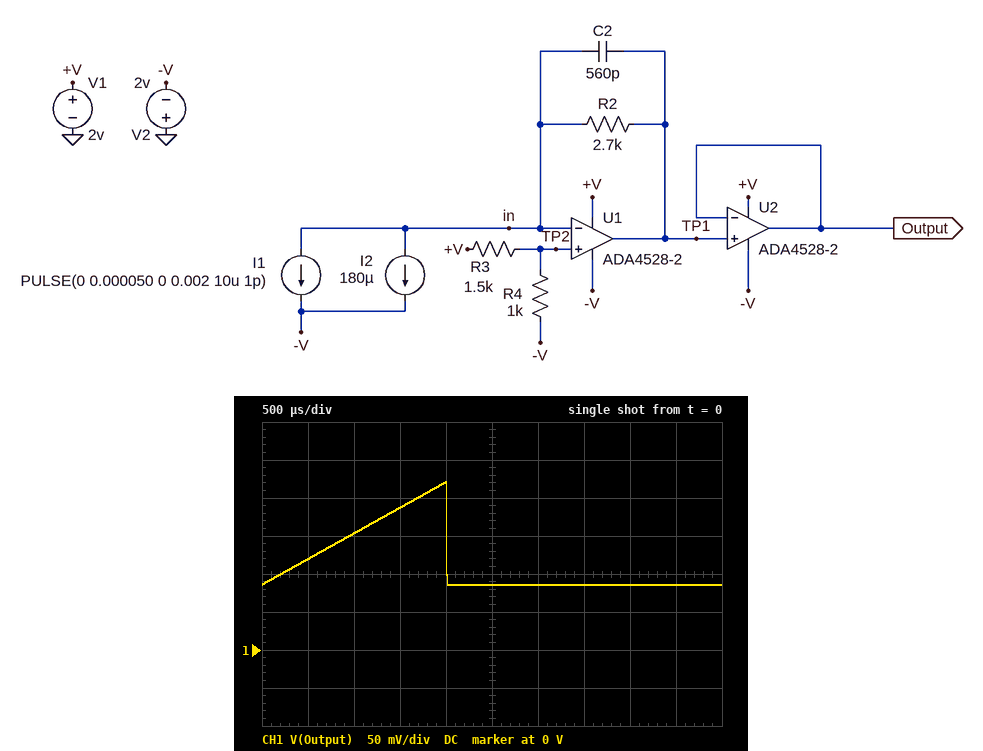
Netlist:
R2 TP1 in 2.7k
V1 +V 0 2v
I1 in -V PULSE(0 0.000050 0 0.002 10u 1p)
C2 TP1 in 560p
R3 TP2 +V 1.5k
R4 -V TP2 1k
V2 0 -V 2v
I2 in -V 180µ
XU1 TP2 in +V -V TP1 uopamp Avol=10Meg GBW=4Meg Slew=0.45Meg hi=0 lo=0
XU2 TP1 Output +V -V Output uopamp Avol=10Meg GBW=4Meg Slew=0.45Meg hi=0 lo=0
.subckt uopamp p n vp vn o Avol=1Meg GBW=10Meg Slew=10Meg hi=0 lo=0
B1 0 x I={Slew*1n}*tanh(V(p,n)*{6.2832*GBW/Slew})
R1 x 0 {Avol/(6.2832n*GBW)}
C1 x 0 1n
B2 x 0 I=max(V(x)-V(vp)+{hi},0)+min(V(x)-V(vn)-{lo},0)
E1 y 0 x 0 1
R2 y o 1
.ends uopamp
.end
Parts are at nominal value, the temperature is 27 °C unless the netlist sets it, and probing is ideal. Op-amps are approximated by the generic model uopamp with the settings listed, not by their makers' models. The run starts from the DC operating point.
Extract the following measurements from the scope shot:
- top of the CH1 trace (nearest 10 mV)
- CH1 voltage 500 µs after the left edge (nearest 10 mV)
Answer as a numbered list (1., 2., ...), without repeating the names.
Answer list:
1. 220 mV
2. 120 mV
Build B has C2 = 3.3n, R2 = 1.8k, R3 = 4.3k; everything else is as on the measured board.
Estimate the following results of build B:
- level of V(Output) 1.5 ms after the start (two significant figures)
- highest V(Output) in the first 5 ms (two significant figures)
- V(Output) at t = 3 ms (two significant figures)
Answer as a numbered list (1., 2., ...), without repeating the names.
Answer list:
1. -850 mV
2. -830 mV
3. -920 mV
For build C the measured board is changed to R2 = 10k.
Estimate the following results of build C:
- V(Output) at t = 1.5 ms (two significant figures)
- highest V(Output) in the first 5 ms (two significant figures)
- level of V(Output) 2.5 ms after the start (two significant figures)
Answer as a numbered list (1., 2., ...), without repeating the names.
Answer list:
1. 1.8 V
2. 1.9 V
3. 1.4 V
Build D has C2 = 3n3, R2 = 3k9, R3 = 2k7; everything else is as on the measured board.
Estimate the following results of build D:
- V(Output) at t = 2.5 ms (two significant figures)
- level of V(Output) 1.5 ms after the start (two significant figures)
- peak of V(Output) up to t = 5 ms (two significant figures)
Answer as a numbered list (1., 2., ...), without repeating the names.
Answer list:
1. -220 mV
2. -72 mV
3. -23 mV
